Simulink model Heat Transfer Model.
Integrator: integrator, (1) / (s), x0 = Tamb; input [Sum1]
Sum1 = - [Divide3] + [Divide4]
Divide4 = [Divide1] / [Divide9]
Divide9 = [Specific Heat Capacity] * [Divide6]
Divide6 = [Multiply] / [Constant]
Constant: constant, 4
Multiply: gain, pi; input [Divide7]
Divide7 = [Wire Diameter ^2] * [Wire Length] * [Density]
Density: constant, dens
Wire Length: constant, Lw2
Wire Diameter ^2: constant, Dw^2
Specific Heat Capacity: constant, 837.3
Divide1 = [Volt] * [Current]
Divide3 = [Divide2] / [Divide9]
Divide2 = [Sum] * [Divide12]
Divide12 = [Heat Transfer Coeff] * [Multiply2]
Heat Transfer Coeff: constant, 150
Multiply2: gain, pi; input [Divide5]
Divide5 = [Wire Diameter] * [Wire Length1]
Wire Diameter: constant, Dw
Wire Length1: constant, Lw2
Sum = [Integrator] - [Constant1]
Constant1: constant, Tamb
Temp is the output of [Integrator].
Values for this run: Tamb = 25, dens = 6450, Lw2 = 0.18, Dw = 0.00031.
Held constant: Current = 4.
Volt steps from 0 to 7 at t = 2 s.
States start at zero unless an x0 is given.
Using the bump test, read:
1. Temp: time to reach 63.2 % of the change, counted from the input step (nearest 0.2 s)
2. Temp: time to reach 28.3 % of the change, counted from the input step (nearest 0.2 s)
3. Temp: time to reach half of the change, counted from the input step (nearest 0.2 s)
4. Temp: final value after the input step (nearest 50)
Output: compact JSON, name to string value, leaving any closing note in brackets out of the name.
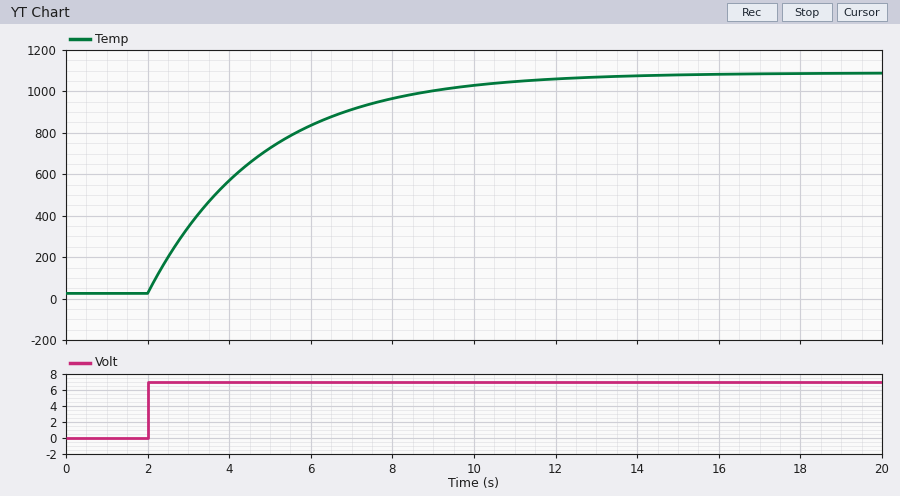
{"Temp: time to reach 63.2 % of the change, counted from the input step": "2.8 s", "Temp: time to reach 28.3 % of the change, counted from the input step": "1.0 s", "Temp: time to reach half of the change, counted from the input step": "2.0 s", "Temp: final value after the input step": "1100"}
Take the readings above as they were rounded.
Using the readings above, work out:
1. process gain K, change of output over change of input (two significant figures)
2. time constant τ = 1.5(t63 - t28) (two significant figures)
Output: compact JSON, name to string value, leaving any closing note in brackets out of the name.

{"process gain K, change of output over change of input": "160", "time constant τ = 1.5(t63 - t28)": "2.7 s"}
